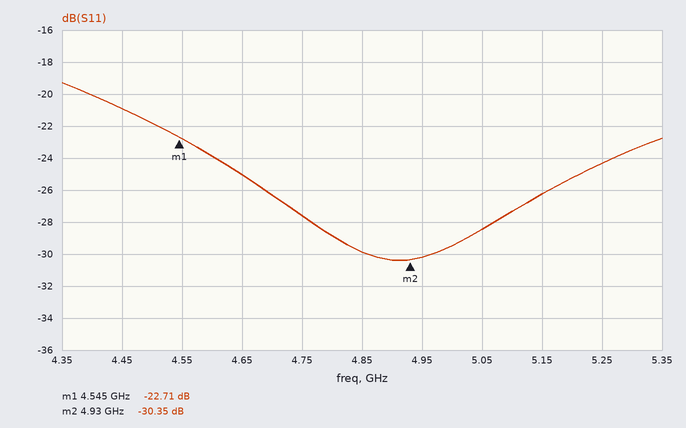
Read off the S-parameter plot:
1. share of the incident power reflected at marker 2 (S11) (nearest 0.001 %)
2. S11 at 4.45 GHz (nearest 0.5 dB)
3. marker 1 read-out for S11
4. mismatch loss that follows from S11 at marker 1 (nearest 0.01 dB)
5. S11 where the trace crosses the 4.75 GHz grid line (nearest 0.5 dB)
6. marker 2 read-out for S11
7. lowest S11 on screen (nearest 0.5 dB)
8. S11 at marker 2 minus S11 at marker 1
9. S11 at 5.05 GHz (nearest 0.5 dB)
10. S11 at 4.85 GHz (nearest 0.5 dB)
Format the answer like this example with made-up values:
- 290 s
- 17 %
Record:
- 0.092 %
- -21.0 dB
- -22.71 dB
- 0.02 dB
- -27.5 dB
- -30.35 dB
- -30.5 dB
- -7.64 dB
- -28.5 dB
- -30.0 dB
